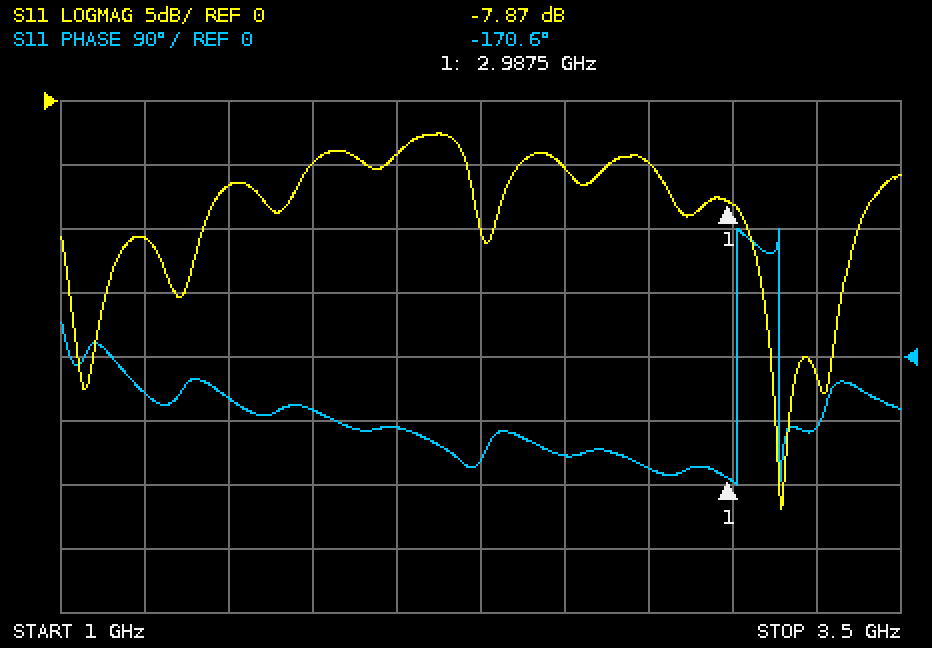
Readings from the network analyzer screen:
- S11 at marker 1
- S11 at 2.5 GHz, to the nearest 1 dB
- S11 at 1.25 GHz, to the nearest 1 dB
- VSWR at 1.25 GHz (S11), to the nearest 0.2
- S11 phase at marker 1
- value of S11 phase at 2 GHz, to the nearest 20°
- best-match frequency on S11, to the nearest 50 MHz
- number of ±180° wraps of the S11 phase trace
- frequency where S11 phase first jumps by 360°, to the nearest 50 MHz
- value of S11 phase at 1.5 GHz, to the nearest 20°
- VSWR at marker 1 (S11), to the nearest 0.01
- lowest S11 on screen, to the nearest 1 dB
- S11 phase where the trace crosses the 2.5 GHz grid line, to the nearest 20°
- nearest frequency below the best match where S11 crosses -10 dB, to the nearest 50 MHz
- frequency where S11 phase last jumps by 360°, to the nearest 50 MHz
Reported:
-7.87 dB
-5 dB
-11 dB
1.8
-170.6°
-100°
3.15 GHz
2
3.00 GHz
-60°
2.36
-32 dB
-140°
3.05 GHz
3.15 GHz
